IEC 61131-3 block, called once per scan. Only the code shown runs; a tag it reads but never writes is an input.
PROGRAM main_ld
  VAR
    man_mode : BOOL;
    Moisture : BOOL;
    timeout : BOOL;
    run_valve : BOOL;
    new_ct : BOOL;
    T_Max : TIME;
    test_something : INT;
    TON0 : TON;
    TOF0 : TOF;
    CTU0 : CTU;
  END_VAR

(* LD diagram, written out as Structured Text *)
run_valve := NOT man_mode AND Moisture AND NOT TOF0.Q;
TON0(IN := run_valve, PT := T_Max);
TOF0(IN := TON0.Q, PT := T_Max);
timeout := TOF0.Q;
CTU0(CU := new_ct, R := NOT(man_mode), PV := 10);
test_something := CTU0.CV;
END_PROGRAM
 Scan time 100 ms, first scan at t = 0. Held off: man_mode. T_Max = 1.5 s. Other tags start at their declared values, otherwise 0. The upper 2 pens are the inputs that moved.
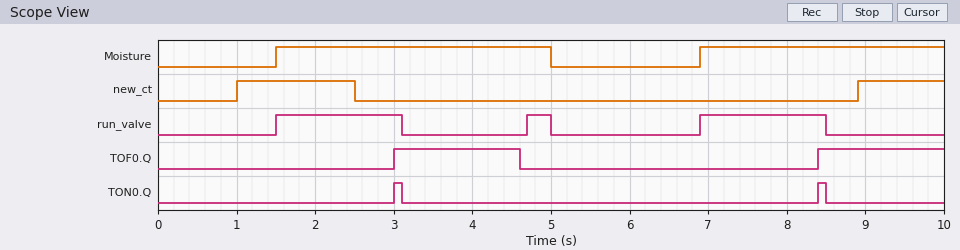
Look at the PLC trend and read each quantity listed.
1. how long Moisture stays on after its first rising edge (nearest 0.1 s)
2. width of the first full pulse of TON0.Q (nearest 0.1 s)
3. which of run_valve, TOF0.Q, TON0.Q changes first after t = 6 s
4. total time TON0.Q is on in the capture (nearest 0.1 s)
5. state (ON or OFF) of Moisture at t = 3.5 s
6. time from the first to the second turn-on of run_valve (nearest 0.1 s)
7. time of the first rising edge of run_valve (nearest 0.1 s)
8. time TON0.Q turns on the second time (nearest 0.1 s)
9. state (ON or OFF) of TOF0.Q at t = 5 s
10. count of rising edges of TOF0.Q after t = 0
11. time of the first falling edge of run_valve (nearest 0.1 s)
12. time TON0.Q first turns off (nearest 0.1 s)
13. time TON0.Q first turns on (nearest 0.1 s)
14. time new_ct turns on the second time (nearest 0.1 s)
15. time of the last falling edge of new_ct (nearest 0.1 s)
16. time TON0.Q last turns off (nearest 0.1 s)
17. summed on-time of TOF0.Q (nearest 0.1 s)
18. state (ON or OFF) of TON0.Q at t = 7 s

3.5 s
0.1 s
run_valve
0.2 s
ON
3.2 s
1.5 s
8.4 s
OFF
2
3.1 s
3.1 s
3.0 s
8.9 s
2.5 s
8.5 s
3.2 s
OFF
